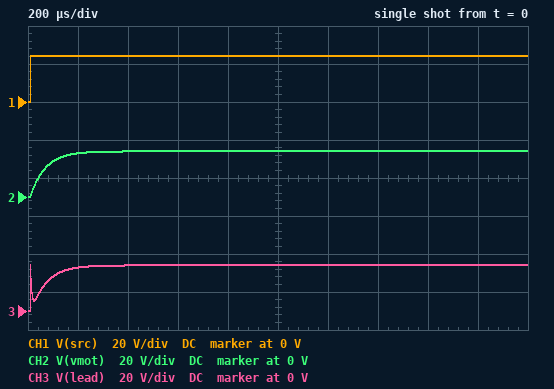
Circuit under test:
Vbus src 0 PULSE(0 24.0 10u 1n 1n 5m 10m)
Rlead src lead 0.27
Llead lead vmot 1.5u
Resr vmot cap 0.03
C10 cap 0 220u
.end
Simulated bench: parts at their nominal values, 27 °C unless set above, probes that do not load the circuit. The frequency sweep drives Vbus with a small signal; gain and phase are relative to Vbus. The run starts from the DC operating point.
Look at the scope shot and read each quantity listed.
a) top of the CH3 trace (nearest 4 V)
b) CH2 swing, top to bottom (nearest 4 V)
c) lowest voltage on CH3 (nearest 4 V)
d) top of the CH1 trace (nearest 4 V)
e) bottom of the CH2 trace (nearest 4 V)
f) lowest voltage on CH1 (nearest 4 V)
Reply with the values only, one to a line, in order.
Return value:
24 V
24 V
0 V
24 V
0 V
0 V
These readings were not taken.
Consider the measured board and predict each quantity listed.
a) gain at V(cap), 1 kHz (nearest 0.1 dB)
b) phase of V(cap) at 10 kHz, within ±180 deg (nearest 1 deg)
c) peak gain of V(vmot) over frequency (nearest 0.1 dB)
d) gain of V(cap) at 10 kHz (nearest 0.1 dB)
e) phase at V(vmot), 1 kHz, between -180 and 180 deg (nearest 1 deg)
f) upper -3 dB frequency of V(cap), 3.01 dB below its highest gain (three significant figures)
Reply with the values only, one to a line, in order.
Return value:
-0.6 dB
-94 deg
0 dB
-12.4 dB
-20 deg
2.61 kHz
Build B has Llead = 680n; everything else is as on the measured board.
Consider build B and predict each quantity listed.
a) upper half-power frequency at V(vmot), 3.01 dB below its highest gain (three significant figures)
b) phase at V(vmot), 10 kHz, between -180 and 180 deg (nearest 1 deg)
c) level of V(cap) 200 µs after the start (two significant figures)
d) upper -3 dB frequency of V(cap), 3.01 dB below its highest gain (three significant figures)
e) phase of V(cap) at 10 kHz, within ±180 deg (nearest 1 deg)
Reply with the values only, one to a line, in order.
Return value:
2.52 kHz
-62 deg
23 V
2.50 kHz
-84 deg
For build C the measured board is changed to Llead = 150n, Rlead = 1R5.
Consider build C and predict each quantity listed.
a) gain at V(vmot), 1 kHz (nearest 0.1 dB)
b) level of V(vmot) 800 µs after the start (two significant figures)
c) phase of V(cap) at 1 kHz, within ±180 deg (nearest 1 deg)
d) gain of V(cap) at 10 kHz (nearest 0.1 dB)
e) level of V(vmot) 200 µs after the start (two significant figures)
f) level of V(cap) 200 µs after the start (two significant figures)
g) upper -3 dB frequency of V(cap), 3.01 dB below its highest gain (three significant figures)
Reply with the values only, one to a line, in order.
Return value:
-7.4 dB
22 V
-65 deg
-26.5 dB
11 V
10 V
473 Hz
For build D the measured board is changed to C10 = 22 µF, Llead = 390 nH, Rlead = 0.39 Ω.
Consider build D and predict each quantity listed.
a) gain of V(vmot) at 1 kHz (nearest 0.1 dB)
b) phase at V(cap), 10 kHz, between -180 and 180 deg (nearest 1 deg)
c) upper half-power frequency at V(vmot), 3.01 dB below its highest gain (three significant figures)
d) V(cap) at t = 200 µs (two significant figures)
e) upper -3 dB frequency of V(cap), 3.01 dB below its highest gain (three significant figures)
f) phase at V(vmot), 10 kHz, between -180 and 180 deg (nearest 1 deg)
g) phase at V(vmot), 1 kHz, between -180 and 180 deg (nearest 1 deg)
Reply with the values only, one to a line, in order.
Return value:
0 dB
-31 deg
19.2 kHz
24 V
19.1 kHz
-29 deg
-3 deg
